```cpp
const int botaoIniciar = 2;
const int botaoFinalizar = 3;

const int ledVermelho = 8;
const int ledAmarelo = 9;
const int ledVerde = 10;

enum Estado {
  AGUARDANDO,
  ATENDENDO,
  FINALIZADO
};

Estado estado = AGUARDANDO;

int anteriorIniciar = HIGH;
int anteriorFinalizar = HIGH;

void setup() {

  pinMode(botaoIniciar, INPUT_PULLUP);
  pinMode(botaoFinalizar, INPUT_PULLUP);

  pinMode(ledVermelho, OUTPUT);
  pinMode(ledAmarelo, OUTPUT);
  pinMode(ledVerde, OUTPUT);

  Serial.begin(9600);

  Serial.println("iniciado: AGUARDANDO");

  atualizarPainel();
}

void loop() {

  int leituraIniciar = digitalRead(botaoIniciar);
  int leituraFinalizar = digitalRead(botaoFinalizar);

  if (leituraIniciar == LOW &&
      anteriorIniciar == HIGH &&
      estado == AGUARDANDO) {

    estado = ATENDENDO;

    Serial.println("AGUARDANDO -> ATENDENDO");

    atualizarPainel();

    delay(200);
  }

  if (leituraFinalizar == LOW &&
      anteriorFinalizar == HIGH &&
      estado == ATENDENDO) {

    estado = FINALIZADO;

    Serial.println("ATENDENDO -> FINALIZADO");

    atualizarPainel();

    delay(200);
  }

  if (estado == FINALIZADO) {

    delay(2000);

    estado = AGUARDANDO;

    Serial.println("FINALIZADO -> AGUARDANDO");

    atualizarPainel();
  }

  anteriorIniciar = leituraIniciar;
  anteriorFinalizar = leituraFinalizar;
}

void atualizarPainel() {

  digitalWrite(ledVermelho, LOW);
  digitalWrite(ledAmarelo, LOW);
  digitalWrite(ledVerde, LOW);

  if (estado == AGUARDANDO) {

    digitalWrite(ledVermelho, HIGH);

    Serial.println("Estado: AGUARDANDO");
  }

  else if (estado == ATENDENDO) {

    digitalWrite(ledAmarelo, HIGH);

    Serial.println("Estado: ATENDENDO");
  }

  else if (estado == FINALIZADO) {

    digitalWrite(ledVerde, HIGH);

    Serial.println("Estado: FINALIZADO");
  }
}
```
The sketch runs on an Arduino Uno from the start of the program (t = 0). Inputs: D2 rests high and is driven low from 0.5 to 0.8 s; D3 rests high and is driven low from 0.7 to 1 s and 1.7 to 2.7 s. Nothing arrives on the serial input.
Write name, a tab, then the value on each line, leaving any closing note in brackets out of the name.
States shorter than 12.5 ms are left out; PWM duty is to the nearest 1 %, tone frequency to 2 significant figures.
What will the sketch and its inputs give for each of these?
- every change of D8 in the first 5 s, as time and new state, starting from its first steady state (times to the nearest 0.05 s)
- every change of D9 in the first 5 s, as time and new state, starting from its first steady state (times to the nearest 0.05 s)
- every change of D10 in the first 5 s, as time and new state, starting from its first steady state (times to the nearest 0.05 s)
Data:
every change of D8 in the first 5 s, as time and new state, starting from its first steady state	0 s high; 0.5 s low; 2.9 s high
every change of D9 in the first 5 s, as time and new state, starting from its first steady state	0 s low; 0.5 s high; 0.7 s low
every change of D10 in the first 5 s, as time and new state, starting from its first steady state	0 s low; 0.7 s high; 2.9 s low
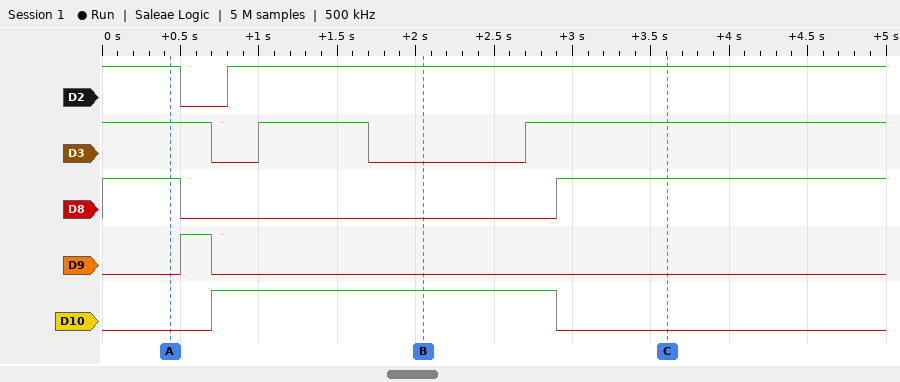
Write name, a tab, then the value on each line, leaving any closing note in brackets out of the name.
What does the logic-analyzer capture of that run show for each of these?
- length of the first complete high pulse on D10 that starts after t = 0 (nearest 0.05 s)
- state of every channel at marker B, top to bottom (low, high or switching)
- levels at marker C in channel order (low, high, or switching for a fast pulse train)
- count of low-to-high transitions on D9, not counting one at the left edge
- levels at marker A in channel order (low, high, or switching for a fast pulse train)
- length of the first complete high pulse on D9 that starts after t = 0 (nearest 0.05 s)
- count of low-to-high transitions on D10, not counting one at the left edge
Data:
length of the first complete high pulse on D10 that starts after t = 0	2.20 s
state of every channel at marker B, top to bottom	D2 high, D3 low, D8 low, D9 low, D10 high
levels at marker C in channel order	D2 high, D3 high, D8 high, D9 low, D10 low
count of low-to-high transitions on D9, not counting one at the left edge	1
levels at marker A in channel order	D2 high, D3 high, D8 high, D9 low, D10 low
length of the first complete high pulse on D9 that starts after t = 0	0.20 s
count of low-to-high transitions on D10, not counting one at the left edge	1
